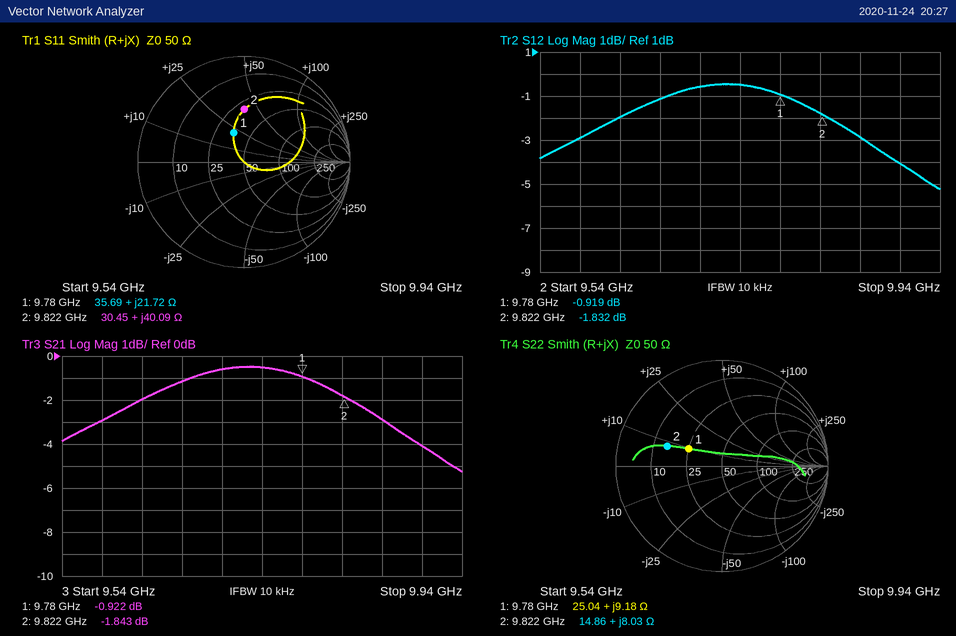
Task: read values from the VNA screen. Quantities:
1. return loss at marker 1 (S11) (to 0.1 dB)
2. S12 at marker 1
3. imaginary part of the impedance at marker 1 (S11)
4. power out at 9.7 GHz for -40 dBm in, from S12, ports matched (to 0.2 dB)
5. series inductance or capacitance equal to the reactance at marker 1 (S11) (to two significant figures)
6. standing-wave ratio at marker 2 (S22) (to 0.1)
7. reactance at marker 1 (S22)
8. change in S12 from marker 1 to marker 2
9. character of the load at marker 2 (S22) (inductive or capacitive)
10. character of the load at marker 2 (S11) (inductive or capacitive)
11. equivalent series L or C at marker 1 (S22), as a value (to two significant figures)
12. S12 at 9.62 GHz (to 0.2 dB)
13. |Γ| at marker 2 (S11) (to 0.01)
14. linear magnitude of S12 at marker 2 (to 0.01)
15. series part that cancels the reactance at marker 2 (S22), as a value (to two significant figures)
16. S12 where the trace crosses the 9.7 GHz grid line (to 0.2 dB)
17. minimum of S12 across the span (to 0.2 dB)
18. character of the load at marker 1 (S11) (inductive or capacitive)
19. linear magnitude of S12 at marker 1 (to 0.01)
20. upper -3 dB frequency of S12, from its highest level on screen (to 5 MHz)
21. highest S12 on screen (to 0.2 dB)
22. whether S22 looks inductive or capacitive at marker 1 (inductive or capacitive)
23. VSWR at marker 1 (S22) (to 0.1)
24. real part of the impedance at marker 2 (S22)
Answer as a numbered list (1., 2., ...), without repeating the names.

1. 10.6 dB
2. -0.919 dB
3. +21.72 Ω
4. -40.6 dBm
5. 350 pH
6. 3.5
7. +9.18 Ω
8. -0.913 dB
9. inductive
10. inductive
11. 150 pH
12. -2.0 dB
13. 0.50
14. 0.81
15. 2.0 pF
16. -0.6 dB
17. -5.2 dB
18. inductive
19. 0.90
20. 9.880 GHz
21. -0.4 dB
22. inductive
23. 2.1
24. 14.86 Ω
